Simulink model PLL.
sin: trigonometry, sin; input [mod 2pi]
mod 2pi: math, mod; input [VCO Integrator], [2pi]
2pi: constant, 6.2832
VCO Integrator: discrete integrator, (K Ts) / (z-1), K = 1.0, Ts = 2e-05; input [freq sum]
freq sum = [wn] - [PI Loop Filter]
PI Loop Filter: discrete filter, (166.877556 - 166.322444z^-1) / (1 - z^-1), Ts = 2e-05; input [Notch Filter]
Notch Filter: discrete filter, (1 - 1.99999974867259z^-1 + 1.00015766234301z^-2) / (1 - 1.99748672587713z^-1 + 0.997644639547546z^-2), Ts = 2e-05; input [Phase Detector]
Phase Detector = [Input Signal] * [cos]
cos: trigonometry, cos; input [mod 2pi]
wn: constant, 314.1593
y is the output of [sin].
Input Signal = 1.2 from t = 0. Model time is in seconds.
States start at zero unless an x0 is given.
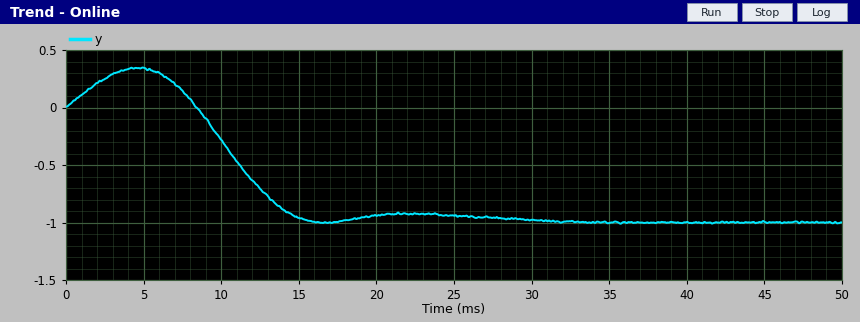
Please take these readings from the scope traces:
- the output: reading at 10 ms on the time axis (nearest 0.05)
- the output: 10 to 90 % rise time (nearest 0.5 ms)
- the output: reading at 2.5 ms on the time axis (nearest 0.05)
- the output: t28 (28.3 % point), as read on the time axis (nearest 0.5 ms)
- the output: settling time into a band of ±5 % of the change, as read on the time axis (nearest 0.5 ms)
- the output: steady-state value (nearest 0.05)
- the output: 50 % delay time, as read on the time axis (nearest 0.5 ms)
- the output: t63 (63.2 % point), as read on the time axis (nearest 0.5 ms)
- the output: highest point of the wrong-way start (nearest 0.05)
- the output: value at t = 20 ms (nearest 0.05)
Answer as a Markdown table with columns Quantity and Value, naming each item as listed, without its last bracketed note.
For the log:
| Quantity | Value |
|---|---|
| the output: reading at 10 ms on the time axis | -0.30 |
| the output: 10 to 90 % rise time | 5.0 ms |
| the output: reading at 2.5 ms on the time axis | 0.25 |
| the output: t28 (28.3 % point), as read on the time axis | 10.0 ms |
| the output: settling time into a band of ±5 % of the change, as read on the time axis | 26.0 ms |
| the output: steady-state value | -1.00 |
| the output: 50 % delay time, as read on the time axis | 11.0 ms |
| the output: t63 (63.2 % point), as read on the time axis | 12.0 ms |
| the output: highest point of the wrong-way start | 0.35 |
| the output: value at t = 20 ms | -0.95 |
